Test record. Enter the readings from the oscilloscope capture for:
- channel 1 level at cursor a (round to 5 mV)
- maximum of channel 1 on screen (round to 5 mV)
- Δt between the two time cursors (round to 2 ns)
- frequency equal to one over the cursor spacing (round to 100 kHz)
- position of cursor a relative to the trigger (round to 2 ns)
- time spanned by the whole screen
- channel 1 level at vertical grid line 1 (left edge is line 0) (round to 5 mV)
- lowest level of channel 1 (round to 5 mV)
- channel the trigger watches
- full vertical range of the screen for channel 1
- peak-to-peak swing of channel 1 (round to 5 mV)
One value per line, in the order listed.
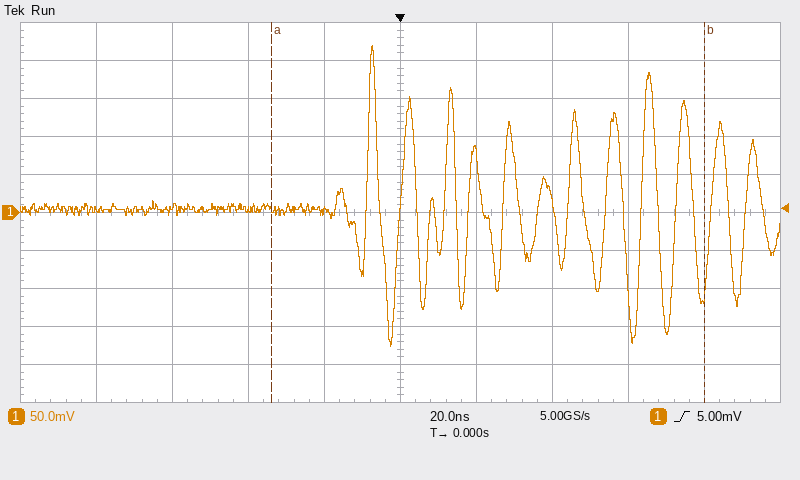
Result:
5 mV
220 mV
114 ns
8.8 MHz
-34 ns
200 ns
5 mV
-175 mV
channel 1
500 mV
395 mV
